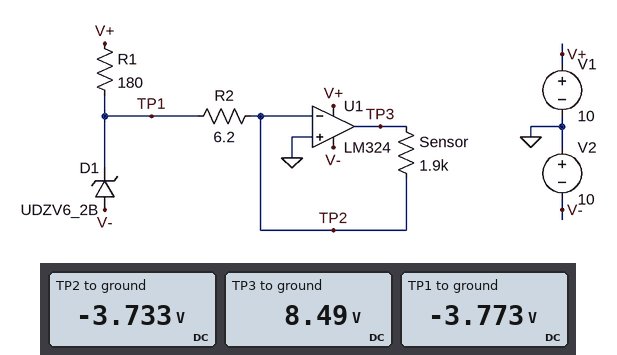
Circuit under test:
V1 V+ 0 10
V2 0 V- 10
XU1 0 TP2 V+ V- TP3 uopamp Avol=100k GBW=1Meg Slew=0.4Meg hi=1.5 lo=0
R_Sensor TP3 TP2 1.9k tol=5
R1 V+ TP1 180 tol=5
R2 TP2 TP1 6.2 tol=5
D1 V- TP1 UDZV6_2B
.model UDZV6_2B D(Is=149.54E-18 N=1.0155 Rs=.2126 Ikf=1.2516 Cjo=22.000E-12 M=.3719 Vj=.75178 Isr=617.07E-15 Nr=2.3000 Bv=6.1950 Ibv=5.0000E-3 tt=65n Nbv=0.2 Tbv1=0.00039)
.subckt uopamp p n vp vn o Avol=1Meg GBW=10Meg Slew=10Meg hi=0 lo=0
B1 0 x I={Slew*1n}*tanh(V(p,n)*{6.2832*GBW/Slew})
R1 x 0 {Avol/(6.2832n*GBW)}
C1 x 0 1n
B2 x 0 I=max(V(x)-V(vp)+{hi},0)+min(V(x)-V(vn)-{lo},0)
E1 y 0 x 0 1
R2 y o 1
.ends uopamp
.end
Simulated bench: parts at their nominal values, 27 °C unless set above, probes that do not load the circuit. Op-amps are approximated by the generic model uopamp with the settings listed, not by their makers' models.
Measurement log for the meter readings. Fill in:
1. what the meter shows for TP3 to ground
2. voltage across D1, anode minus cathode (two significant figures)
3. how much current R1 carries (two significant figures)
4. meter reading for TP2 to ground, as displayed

8.49 V
-6.2 V
77 mA
-3.733 V
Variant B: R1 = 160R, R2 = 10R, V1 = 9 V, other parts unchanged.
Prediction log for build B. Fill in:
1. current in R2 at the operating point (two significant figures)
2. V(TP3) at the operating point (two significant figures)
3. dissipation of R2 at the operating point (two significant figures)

5.9 mA
7.5 V
350 µW
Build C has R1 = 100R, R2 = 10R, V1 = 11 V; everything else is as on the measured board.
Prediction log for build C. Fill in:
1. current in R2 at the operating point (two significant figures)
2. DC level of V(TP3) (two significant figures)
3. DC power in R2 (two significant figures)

6.9 mA
9.5 V
480 µW
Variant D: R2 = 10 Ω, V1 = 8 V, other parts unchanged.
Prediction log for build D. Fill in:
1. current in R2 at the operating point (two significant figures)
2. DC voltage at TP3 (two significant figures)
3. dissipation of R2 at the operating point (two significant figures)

5.4 mA
6.5 V
290 µW
